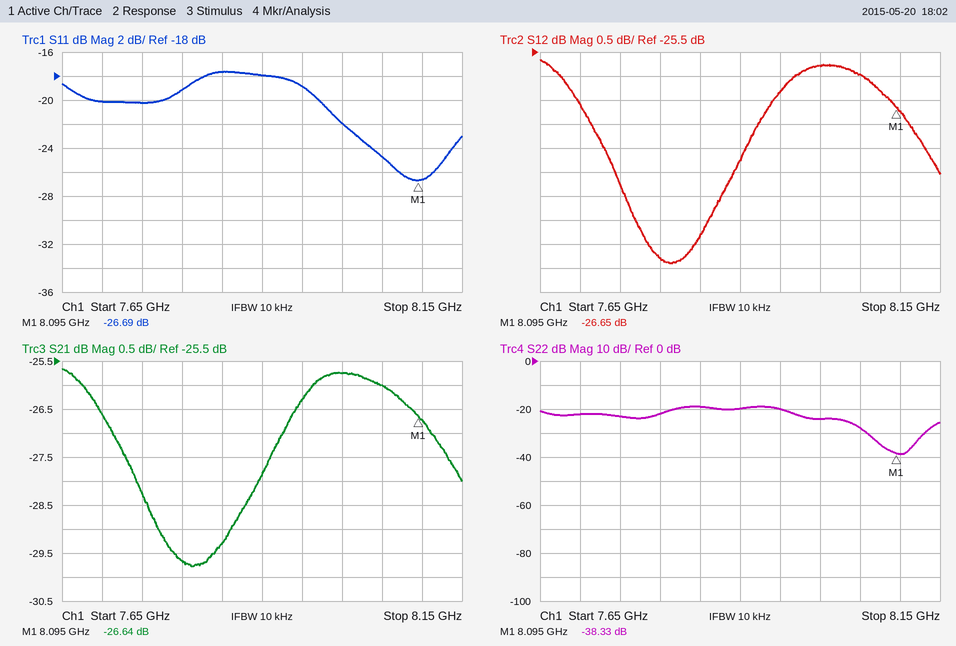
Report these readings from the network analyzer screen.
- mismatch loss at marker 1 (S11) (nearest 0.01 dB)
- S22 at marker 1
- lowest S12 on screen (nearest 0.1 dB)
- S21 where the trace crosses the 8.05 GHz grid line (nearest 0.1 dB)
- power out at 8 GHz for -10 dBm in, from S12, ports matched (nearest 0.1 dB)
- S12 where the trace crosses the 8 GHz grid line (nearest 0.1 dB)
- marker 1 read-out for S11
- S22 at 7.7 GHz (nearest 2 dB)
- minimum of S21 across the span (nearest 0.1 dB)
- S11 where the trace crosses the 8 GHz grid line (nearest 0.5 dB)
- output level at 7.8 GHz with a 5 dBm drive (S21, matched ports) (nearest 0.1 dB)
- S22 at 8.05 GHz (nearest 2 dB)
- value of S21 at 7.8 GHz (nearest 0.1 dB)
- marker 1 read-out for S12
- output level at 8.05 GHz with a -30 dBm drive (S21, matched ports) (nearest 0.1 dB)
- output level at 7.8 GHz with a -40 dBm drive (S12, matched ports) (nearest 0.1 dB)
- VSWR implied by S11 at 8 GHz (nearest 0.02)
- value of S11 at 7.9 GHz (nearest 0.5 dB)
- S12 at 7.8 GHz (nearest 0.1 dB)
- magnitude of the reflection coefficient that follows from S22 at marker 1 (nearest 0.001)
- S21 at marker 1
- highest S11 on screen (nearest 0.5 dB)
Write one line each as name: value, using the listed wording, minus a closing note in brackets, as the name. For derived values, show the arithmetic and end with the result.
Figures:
mismatch loss at marker 1 (S11): −10 log10(1 − 10^(-26.69/10)) ≈ 0.01 dB
S22 at marker 1: -38.33 dB
lowest S12 on screen: -29.9 dB
S21 where the trace crosses the 8.05 GHz grid line: -26.0 dB
power out at 8 GHz for -10 dBm in, from S12, ports matched: -10 dBm + (-25.8 dB) = -35.8 dBm
S12 where the trace crosses the 8 GHz grid line: -25.8 dB
marker 1 read-out for S11: -26.69 dB
S22 at 7.7 GHz: -22 dB
minimum of S21 across the span: -29.8 dB
S11 where the trace crosses the 8 GHz grid line: -22.0 dB
output level at 7.8 GHz with a 5 dBm drive (S21, matched ports): 5 dBm + (-29.7 dB) = -24.7 dBm
S22 at 8.05 GHz: -28 dB
value of S21 at 7.8 GHz: -29.7 dB
marker 1 read-out for S12: -26.65 dB
output level at 8.05 GHz with a -30 dBm drive (S21, matched ports): -30 dBm + (-26.0 dB) = -56.0 dBm
output level at 7.8 GHz with a -40 dBm drive (S12, matched ports): -40 dBm + (-29.8 dB) = -69.8 dBm
VSWR implied by S11 at 8 GHz: |Γ| = 10^(-22/20) = 0.0794; VSWR = (1 + 0.0794)/(1 − 0.0794) ≈ 1.17, so 1.18 to the nearest 0.02
value of S11 at 7.9 GHz: -18.0 dB
S12 at 7.8 GHz: -29.8 dB
magnitude of the reflection coefficient that follows from S22 at marker 1: 10^(-38.33/20) ≈ 0.012
S21 at marker 1: -26.64 dB
highest S11 on screen: -17.5 dB
